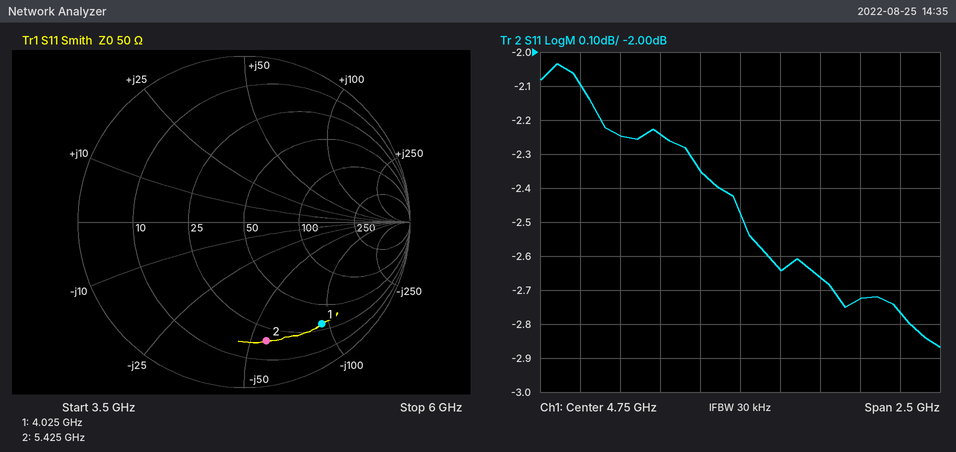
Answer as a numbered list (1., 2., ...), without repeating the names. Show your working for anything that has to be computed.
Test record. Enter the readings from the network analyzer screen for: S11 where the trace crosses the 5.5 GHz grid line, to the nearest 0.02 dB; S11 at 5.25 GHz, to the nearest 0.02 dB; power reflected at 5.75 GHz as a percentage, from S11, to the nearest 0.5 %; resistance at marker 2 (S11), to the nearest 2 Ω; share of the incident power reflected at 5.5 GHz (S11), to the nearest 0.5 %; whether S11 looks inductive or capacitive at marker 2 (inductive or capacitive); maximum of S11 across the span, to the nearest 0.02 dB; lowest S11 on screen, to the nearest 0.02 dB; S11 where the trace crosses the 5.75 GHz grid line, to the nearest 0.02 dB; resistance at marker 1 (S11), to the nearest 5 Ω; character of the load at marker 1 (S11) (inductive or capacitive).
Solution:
1. -2.72 dB
2. -2.66 dB
3. 10^(-2.76/10) ≈ 53.0 %
4. 18 Ω
5. 10^(-2.72/10) ≈ 53.5 %
6. capacitive
7. -2.04 dB
8. -2.86 dB
9. -2.76 dB
10. 30 Ω
11. capacitive
